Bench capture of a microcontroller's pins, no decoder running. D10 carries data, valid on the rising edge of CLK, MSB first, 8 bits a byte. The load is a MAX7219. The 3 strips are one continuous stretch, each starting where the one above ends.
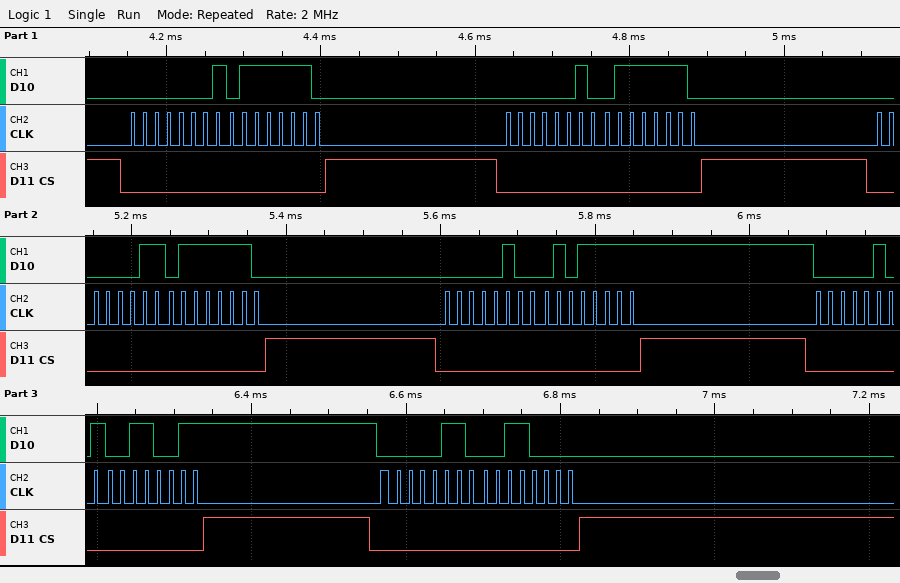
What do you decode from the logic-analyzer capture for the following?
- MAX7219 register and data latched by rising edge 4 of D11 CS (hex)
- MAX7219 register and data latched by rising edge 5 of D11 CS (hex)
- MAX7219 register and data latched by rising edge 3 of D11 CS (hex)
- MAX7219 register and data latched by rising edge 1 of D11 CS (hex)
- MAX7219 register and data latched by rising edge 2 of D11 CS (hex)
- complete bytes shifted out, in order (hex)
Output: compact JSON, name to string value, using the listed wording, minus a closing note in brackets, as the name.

{"MAX7219 register and data latched by rising edge 4 of D11 CS": "register 0x4, data 0x5F", "MAX7219 register and data latched by rising edge 5 of D11 CS": "register 0x5, data 0x33", "MAX7219 register and data latched by rising edge 3 of D11 CS": "register 0x3, data 0x7E", "MAX7219 register and data latched by rising edge 1 of D11 CS": "register 0x1, data 0x7E", "MAX7219 register and data latched by rising edge 2 of D11 CS": "register 0x2, data 0x7E", "complete bytes shifted out, in order": "01 7E 02 7E 03 7E 04 5F 05 33 06 30"}
